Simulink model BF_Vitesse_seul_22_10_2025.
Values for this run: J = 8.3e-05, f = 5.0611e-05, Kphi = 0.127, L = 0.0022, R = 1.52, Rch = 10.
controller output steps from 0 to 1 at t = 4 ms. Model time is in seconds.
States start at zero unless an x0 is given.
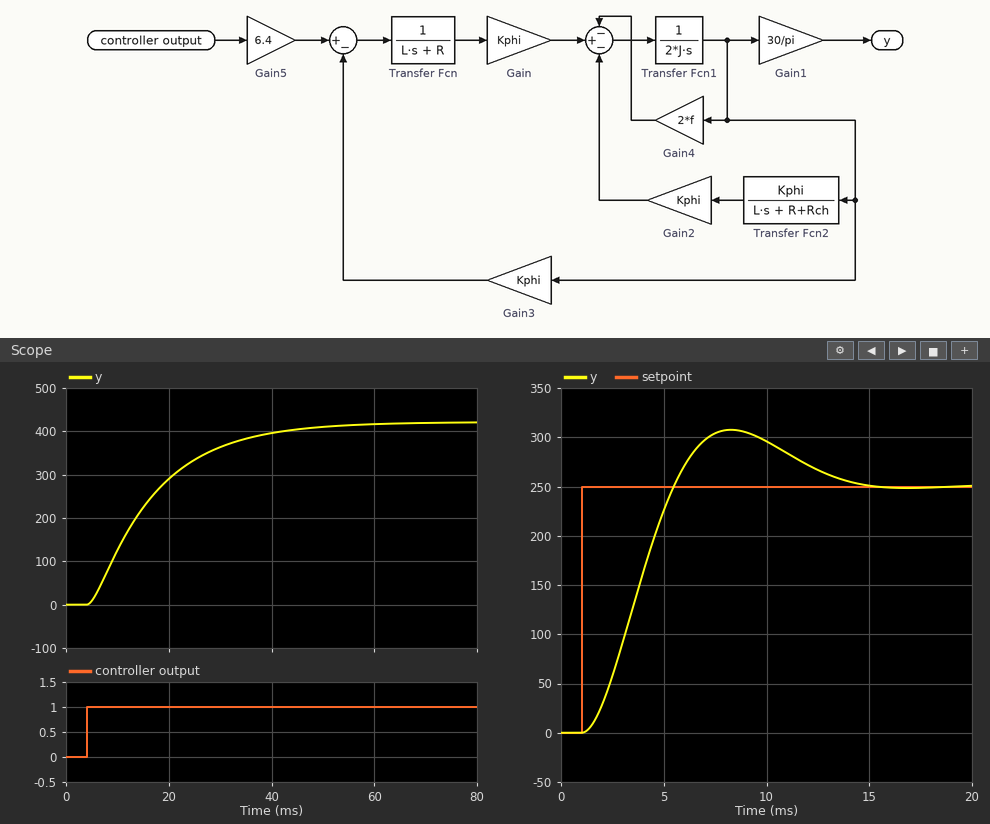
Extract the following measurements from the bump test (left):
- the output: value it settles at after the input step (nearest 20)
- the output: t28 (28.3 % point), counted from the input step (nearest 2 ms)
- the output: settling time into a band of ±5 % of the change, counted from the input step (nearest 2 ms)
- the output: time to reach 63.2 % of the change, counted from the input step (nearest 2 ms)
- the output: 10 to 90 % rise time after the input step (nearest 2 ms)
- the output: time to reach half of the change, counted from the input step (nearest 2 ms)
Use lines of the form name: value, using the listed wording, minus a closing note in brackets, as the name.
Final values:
the output: value it settles at after the input step: 420
the output: t28 (28.3 % point), counted from the input step: 6 ms
the output: settling time into a band of ±5 % of the change, counted from the input step: 38 ms
the output: time to reach 63.2 % of the change, counted from the input step: 14 ms
the output: 10 to 90 % rise time after the input step: 28 ms
the output: time to reach half of the change, counted from the input step: 10 ms
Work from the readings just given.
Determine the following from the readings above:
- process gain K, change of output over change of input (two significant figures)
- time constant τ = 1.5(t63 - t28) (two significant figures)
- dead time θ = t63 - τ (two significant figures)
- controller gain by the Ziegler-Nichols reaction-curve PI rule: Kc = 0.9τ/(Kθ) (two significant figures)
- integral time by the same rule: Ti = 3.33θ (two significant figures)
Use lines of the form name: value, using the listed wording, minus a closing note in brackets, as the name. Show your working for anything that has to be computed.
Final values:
process gain K, change of output over change of input: (420 - 0) / 1 = 420
time constant τ = 1.5(t63 - t28): 1.5 × (14 - 6) = 12 ms
dead time θ = t63 - τ: 14 - 12 = 2.0 ms
controller gain by the Ziegler-Nichols reaction-curve PI rule: Kc = 0.9τ/(Kθ): 0.9 × 12 / (420 × 2) = 0.013
integral time by the same rule: Ti = 3.33θ: 3.33 × 2 = 6.7 ms
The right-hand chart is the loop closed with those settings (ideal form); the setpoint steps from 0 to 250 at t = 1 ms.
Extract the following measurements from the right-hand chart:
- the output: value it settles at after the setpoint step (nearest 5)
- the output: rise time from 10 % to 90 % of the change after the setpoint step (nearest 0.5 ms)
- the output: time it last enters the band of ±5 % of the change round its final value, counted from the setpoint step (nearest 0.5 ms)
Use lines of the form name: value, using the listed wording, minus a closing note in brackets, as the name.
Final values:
the output: value it settles at after the setpoint step: 250
the output: rise time from 10 % to 90 % of the change after the setpoint step: 3.0 ms
the output: time it last enters the band of ±5 % of the change round its final value, counted from the setpoint step: 12.0 ms
